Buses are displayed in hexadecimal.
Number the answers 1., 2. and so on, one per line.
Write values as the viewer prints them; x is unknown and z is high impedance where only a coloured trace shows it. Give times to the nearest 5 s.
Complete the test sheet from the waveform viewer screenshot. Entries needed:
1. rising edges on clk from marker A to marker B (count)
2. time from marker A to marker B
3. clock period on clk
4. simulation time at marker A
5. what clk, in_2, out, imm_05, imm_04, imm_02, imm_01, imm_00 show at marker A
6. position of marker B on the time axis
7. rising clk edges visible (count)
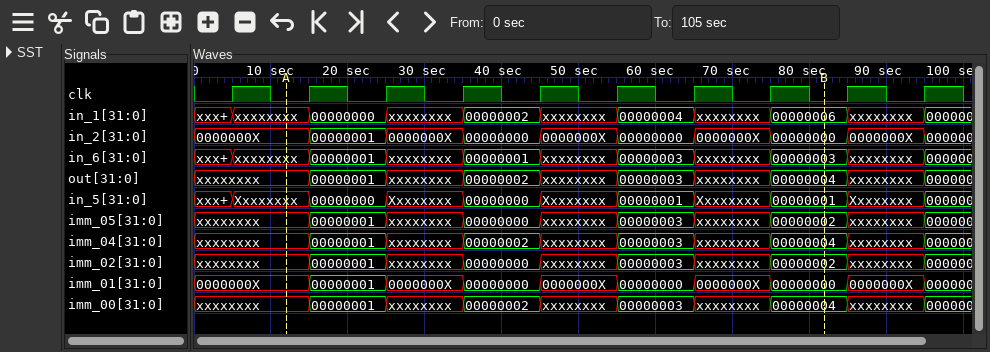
1. 7
2. 70 s
3. 10 s
4. 10 s
5. clk=0, in_2=0000000X, out=xxxxxxxx, imm_05=xxxxxxxx, imm_04=xxxxxxxx, imm_02=xxxxxxxx, imm_01=0000000X, imm_00=xxxxxxxx
6. 80 s
7. 10
